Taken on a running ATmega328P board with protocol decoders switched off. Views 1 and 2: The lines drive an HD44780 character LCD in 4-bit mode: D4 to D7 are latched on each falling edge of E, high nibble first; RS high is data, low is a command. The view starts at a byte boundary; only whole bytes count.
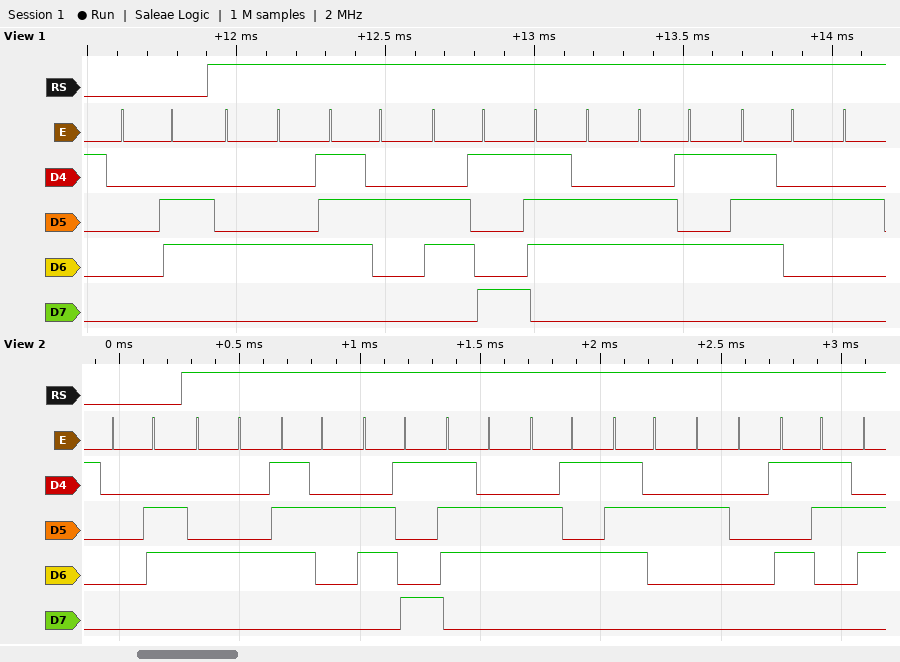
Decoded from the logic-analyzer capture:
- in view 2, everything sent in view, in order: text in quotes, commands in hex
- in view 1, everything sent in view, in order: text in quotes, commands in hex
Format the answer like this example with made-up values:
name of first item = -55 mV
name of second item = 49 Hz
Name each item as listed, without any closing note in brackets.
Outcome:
in view 2, everything sent in view, in order: text in quotes, commands in hex = 0x06 "Driver S"
in view 1, everything sent in view, in order: text in quotes, commands in hex = 0x06 "Driver"
